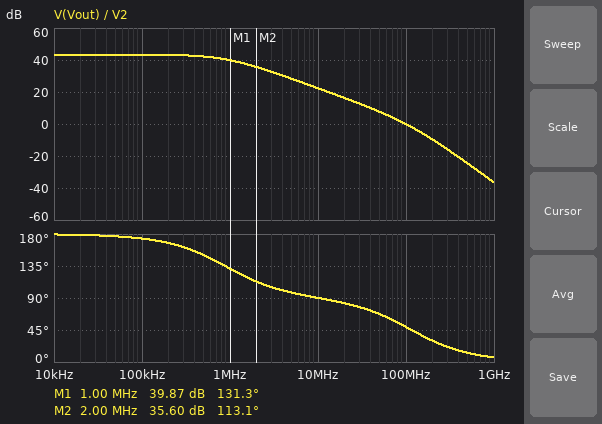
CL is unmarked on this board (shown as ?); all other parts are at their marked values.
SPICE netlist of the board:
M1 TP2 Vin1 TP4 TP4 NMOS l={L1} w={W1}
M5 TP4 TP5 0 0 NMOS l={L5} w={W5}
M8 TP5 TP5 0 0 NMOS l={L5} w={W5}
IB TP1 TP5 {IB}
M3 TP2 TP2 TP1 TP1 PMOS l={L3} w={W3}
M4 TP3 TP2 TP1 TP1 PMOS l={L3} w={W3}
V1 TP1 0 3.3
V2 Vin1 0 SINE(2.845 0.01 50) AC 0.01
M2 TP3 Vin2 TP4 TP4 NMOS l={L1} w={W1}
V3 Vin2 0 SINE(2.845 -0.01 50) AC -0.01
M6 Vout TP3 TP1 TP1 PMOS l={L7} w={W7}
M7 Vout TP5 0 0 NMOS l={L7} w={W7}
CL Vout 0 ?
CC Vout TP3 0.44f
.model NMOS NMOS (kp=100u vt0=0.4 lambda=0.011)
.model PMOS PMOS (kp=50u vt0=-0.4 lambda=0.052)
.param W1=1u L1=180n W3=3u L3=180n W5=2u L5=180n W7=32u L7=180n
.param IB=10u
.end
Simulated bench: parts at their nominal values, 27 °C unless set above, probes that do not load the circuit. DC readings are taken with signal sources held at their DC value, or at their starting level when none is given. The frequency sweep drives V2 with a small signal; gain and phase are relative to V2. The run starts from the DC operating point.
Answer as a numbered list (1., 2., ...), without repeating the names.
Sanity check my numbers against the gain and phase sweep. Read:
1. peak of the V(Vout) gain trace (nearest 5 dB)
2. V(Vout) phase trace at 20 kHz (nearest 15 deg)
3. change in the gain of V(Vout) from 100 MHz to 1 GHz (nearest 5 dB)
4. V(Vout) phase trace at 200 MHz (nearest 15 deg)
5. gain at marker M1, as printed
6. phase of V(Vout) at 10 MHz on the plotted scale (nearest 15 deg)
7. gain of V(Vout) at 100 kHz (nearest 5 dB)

1. 45 dB
2. 180 deg
3. -35 dB
4. 30 deg
5. 39.87 dB
6. 90 deg
7. 45 dB
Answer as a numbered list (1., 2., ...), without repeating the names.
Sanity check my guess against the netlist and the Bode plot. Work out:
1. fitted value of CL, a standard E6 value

1. 330 pF
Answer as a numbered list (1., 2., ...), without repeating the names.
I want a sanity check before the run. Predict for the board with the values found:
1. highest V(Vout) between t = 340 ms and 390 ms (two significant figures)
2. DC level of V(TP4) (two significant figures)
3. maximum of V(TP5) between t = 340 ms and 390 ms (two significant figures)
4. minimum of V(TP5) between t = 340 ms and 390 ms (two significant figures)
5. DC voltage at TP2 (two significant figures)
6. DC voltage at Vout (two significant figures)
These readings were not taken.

1. 3.3 V
2. 2.3 V
3. 530 mV
4. 530 mV
5. 2.8 V
6. 29 mV
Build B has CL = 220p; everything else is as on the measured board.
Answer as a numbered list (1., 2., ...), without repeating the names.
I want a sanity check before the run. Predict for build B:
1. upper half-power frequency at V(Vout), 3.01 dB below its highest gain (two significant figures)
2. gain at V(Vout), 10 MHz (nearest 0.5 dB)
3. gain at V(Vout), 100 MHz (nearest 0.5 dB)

1. 1.3 MHz
2. 26.0 dB
3. 3.5 dB
